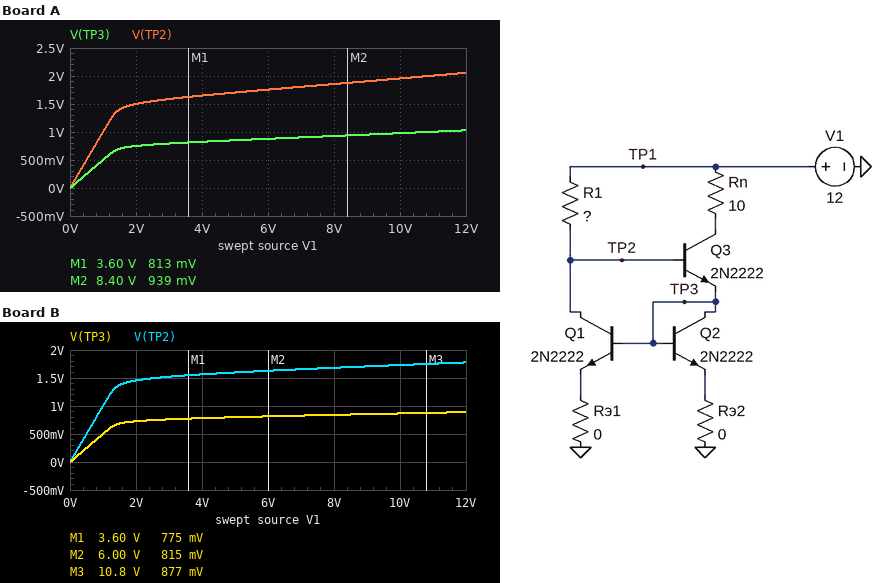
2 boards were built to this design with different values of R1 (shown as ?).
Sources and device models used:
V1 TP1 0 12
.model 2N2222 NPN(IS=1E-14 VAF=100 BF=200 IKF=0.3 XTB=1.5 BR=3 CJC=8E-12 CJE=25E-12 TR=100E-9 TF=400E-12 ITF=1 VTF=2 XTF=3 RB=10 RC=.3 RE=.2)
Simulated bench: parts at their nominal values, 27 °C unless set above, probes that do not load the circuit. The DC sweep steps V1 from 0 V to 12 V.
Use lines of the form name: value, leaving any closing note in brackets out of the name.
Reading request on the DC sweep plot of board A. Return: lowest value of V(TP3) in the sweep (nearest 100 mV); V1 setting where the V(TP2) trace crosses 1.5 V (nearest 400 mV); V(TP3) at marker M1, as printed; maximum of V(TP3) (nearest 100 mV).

lowest value of V(TP3) in the sweep: 0 V
V1 setting where the V(TP2) trace crosses 1.5 V: 2.0 V
V(TP3) at marker M1, as printed: 813 mV
maximum of V(TP3): 1.0 V
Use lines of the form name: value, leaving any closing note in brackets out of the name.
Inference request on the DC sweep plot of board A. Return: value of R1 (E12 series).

value of R1: 18 Ω
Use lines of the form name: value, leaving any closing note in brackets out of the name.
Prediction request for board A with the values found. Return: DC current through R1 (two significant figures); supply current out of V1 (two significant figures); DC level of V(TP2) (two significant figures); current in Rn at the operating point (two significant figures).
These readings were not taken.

DC current through R1: 550 mA
supply current out of V1: 1.1 A
DC level of V(TP2): 2.1 V
current in Rn at the operating point: 550 mA
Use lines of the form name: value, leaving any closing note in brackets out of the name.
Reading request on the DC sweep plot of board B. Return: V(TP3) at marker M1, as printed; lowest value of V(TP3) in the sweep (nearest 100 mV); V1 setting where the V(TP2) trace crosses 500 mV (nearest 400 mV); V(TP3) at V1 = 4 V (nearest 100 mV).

V(TP3) at marker M1, as printed: 775 mV
lowest value of V(TP3) in the sweep: 0 V
V1 setting where the V(TP2) trace crosses 500 mV: 400 mV
V(TP3) at V1 = 4 V: 800 mV
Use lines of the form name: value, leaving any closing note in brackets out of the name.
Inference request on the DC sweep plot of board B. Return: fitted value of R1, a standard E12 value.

fitted value of R1, a standard E12 value: 39 Ω
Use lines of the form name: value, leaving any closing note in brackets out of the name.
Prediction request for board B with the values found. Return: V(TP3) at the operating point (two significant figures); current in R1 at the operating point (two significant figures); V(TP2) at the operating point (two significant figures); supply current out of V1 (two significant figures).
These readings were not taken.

V(TP3) at the operating point: 890 mV
current in R1 at the operating point: 260 mA
V(TP2) at the operating point: 1.8 V
supply current out of V1: 520 mA
